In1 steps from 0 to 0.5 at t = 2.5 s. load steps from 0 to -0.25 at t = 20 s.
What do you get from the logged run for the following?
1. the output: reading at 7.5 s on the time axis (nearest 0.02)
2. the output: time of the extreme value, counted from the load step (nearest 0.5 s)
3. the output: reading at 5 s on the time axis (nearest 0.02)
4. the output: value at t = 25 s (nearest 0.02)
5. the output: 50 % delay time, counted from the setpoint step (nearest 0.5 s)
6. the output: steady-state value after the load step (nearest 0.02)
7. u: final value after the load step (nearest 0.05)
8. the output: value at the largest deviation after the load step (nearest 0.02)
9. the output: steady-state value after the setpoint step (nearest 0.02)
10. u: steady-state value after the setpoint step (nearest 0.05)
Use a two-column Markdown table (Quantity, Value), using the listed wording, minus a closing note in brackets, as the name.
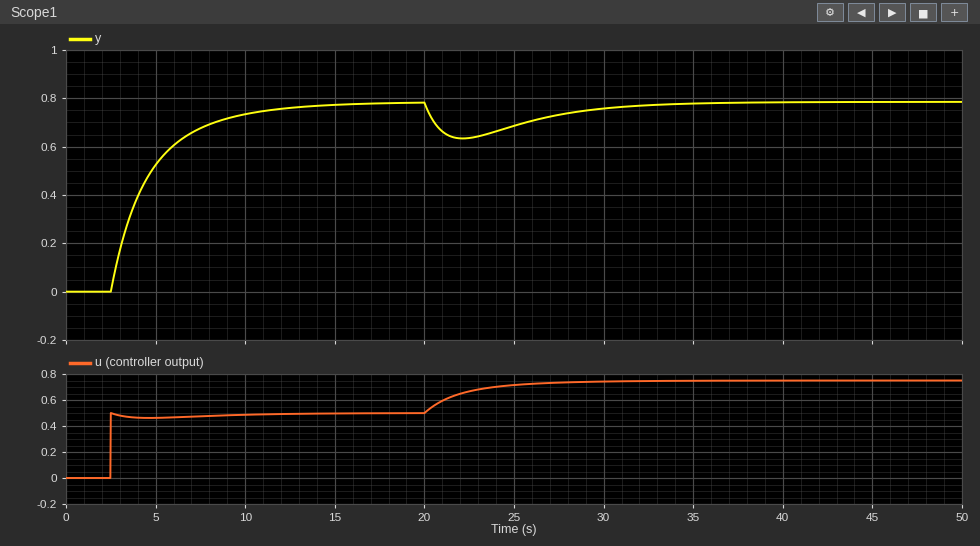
| Quantity | Value |
|---|---|
| the output: reading at 7.5 s on the time axis | 0.68 |
| the output: time of the extreme value, counted from the load step | 2.0 s |
| the output: reading at 5 s on the time axis | 0.52 |
| the output: value at t = 25 s | 0.68 |
| the output: 50 % delay time, counted from the setpoint step | 1.5 s |
| the output: steady-state value after the load step | 0.78 |
| u: final value after the load step | 0.75 |
| the output: value at the largest deviation after the load step | 0.64 |
| the output: steady-state value after the setpoint step | 0.78 |
| u: steady-state value after the setpoint step | 0.50 |
